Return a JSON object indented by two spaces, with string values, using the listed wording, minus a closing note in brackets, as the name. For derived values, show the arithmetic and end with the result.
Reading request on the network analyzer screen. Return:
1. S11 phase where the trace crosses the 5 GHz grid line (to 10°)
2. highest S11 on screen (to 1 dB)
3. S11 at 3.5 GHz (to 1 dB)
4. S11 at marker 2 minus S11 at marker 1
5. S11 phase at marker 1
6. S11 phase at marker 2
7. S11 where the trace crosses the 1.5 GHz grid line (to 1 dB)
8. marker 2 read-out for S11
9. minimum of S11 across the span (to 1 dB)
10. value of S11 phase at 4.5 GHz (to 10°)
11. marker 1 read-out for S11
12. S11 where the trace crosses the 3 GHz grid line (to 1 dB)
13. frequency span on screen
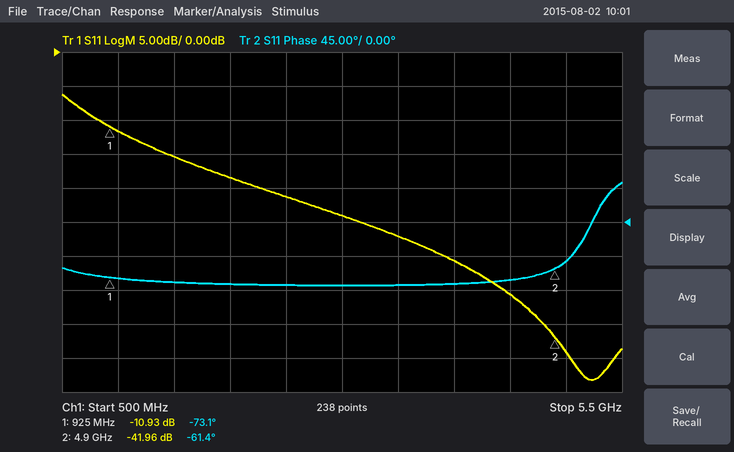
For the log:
{
  "S11 phase where the trace crosses the 5 GHz grid line": "-50°",
  "highest S11 on screen": "-6 dB",
  "S11 at 3.5 GHz": "-27 dB",
  "S11 at marker 2 minus S11 at marker 1": "-41.96 − (-10.93) = -31.03 dB",
  "S11 phase at marker 1": "-73.1°",
  "S11 phase at marker 2": "-61.4°",
  "S11 where the trace crosses the 1.5 GHz grid line": "-15 dB",
  "marker 2 read-out for S11": "-41.96 dB",
  "minimum of S11 across the span": "-48 dB",
  "value of S11 phase at 4.5 GHz": "-80°",
  "marker 1 read-out for S11": "-10.93 dB",
  "S11 where the trace crosses the 3 GHz grid line": "-24 dB",
  "frequency span on screen": "5 GHz"
}
